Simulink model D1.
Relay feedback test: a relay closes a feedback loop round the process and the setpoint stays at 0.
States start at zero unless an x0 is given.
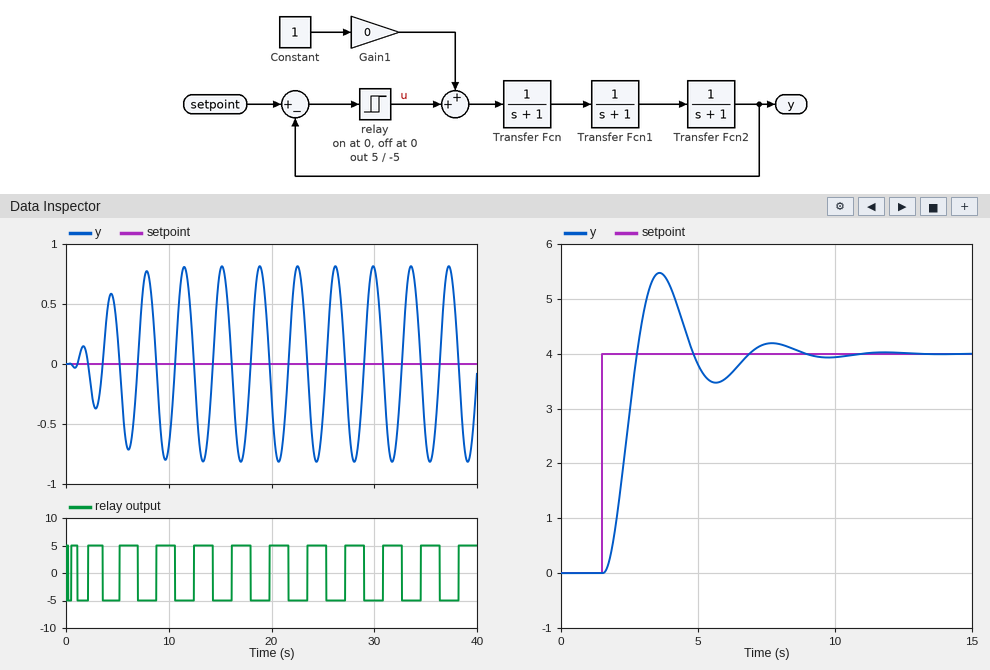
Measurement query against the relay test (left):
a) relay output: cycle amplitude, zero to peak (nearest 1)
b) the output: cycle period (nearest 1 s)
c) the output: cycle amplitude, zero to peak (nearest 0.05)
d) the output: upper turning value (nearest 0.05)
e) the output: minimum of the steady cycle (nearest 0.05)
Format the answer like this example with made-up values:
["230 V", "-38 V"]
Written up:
["5", "4 s", "0.80", "0.80", "-0.80"]
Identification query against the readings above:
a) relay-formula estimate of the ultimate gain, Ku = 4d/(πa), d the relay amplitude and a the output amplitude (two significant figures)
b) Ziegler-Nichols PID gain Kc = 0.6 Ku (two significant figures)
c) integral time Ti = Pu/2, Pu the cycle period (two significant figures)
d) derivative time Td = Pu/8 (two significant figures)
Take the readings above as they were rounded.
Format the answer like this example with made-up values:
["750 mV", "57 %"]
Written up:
["8.0", "4.8", "2.0 s", "0.50 s"]
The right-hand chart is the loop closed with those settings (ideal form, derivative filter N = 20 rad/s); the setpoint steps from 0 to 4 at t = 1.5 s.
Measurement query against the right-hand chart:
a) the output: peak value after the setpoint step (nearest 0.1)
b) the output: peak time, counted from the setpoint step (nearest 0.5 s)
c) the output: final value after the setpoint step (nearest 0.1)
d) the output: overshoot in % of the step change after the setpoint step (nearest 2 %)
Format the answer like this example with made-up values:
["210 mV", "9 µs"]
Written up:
["5.5", "2.0 s", "4.0", "36 %"]
